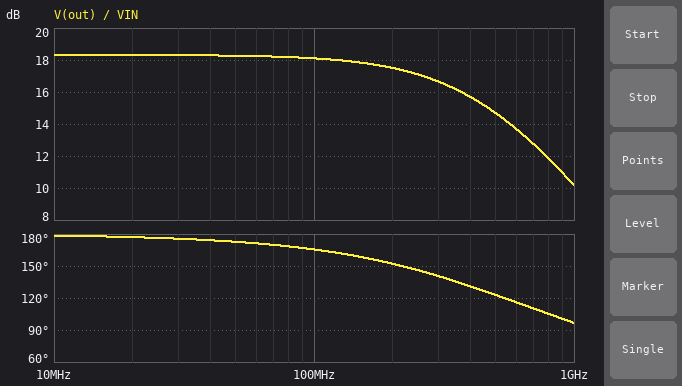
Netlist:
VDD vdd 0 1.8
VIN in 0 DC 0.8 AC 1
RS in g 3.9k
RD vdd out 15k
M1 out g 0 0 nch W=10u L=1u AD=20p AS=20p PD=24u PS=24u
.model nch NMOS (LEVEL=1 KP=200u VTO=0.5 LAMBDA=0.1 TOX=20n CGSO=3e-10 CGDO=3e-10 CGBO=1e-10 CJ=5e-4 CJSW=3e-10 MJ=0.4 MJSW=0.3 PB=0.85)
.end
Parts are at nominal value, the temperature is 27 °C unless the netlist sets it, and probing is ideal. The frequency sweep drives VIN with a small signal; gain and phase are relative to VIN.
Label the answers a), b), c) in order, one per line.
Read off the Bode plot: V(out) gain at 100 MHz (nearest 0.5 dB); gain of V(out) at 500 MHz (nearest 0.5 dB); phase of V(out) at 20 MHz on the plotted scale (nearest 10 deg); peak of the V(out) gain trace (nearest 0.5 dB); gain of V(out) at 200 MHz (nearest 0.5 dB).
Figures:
a) 18.0 dB
b) 14.5 dB
c) 180 deg
d) 18.5 dB
e) 17.5 dB
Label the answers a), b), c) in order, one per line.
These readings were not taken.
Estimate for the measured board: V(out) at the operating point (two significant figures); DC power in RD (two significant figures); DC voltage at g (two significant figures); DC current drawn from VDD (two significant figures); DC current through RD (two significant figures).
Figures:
a) 400 mV
b) 130 µW
c) 800 mV
d) 94 µA
e) 94 µA
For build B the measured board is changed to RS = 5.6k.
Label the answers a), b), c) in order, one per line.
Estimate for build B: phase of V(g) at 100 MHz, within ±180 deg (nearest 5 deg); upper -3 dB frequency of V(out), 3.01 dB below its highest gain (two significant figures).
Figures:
a) -10 deg
b) 370 MHz
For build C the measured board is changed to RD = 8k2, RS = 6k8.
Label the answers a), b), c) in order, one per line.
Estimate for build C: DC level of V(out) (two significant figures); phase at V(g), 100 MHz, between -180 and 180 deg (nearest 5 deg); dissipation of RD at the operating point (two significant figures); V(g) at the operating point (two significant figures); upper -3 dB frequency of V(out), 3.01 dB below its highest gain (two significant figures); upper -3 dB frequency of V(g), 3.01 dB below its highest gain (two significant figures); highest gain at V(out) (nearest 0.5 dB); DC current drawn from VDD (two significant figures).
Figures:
a) 990 mV
b) -10 deg
c) 80 µW
d) 800 mV
e) 520 MHz
f) 630 MHz
g) 14.0 dB
h) 99 µA
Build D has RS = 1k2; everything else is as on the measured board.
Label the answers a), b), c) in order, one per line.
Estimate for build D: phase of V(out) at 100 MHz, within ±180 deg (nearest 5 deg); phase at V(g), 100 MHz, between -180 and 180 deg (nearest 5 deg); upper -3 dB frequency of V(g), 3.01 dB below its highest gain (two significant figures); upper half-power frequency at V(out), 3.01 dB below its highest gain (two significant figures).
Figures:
a) 170 deg
b) 0 deg
c) 6.5 GHz
d) 590 MHz
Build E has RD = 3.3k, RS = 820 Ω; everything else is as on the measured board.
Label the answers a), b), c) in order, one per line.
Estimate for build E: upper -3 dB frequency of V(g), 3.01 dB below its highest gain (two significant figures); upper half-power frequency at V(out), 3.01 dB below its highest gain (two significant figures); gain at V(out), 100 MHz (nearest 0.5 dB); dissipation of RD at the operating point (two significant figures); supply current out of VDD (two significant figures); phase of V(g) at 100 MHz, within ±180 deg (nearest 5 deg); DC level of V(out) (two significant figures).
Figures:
a) 9.6 GHz
b) 2.7 GHz
c) 7.0 dB
d) 35 µW
e) 100 µA
f) 0 deg
g) 1.5 V
